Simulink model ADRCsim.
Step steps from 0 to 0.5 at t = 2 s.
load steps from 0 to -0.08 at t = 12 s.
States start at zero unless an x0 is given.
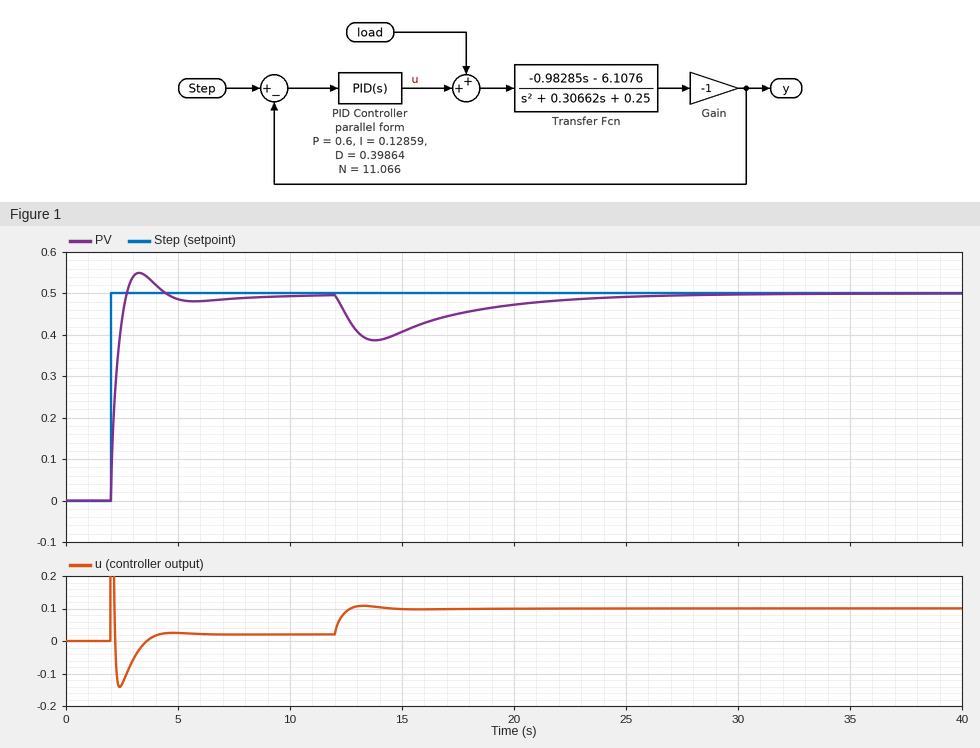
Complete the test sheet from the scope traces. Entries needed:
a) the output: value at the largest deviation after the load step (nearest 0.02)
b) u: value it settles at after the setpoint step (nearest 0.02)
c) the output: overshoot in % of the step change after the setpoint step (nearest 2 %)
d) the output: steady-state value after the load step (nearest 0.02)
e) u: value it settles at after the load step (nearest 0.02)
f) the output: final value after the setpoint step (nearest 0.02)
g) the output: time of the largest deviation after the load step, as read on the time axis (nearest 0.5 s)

0.38
0.02
10 %
0.50
0.10
0.50
14.0 s
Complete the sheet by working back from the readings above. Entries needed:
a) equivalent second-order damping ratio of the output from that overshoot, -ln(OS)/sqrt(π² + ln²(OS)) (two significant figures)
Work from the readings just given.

0.59
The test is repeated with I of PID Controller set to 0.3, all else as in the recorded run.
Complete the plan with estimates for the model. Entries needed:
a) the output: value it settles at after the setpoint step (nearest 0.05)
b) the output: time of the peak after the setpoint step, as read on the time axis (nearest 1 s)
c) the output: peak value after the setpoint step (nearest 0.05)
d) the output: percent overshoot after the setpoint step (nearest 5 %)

0.50
3 s
0.55
15 %
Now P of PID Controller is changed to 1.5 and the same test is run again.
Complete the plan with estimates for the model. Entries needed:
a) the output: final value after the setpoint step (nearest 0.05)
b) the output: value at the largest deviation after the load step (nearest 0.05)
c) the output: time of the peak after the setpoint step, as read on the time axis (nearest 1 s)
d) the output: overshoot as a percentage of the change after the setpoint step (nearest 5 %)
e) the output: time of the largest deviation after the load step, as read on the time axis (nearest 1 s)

0.50
0.45
3 s
15 %
13 s
